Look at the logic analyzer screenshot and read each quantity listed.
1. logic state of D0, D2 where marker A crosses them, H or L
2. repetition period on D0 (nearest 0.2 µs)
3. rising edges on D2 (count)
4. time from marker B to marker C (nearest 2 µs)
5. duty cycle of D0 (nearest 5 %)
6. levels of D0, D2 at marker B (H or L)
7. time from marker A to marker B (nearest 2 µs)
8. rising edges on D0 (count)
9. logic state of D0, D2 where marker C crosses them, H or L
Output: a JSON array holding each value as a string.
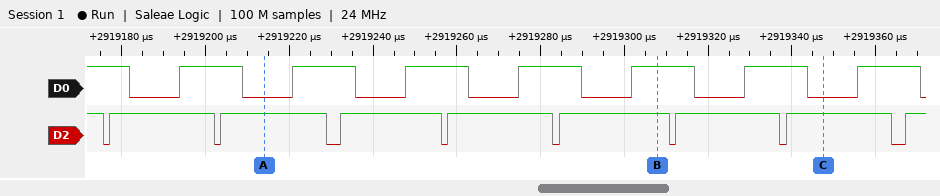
["D0=L, D2=H", "27 µs", "8", "40 µs", "55 %", "D0=H, D2=H", "94 µs", "7", "D0=L, D2=H"]
